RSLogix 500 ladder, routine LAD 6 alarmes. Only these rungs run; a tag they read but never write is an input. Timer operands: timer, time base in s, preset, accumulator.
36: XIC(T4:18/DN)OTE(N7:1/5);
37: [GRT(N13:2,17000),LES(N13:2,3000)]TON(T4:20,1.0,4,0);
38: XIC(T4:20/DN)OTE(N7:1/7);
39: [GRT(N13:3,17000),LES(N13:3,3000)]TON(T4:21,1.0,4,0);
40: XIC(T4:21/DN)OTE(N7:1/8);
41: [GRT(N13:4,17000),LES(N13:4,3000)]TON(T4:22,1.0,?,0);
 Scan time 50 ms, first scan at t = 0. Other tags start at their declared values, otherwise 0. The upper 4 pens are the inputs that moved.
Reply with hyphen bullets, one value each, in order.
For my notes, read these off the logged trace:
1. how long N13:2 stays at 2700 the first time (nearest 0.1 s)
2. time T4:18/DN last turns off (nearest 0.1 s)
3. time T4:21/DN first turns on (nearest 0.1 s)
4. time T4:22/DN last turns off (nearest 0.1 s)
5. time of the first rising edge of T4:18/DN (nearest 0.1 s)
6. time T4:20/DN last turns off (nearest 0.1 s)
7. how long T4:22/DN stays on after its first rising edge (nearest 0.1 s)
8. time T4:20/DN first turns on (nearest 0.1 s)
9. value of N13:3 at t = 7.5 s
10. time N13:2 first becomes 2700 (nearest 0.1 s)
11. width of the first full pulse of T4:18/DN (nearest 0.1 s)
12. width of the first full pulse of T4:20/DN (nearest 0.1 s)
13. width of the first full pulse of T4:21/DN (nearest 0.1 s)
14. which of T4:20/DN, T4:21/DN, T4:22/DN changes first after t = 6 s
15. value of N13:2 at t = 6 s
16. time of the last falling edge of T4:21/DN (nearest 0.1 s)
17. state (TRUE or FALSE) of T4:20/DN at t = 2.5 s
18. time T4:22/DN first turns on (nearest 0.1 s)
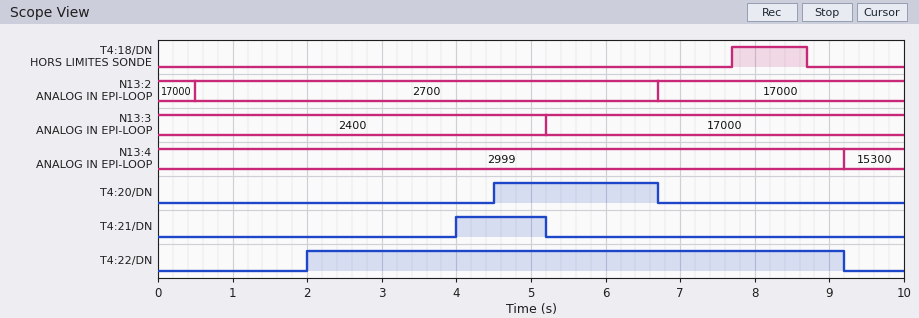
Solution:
- 6.2 s
- 8.7 s
- 4.0 s
- 9.2 s
- 7.7 s
- 6.7 s
- 7.2 s
- 4.5 s
- 17000
- 0.5 s
- 1.0 s
- 2.2 s
- 1.2 s
- T4:20/DN
- 2700
- 5.2 s
- FALSE
- 2.0 s
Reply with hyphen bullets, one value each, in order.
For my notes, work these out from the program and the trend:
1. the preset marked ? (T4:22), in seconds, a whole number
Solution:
- 2 s
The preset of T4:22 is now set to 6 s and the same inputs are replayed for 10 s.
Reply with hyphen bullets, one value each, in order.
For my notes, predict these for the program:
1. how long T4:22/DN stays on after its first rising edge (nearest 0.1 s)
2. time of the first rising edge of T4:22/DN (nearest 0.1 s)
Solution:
- 3.2 s
- 6.0 s
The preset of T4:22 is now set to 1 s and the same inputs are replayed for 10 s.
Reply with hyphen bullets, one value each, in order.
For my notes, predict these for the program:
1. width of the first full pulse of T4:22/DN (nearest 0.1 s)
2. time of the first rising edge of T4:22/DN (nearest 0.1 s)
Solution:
- 8.2 s
- 1.0 s
